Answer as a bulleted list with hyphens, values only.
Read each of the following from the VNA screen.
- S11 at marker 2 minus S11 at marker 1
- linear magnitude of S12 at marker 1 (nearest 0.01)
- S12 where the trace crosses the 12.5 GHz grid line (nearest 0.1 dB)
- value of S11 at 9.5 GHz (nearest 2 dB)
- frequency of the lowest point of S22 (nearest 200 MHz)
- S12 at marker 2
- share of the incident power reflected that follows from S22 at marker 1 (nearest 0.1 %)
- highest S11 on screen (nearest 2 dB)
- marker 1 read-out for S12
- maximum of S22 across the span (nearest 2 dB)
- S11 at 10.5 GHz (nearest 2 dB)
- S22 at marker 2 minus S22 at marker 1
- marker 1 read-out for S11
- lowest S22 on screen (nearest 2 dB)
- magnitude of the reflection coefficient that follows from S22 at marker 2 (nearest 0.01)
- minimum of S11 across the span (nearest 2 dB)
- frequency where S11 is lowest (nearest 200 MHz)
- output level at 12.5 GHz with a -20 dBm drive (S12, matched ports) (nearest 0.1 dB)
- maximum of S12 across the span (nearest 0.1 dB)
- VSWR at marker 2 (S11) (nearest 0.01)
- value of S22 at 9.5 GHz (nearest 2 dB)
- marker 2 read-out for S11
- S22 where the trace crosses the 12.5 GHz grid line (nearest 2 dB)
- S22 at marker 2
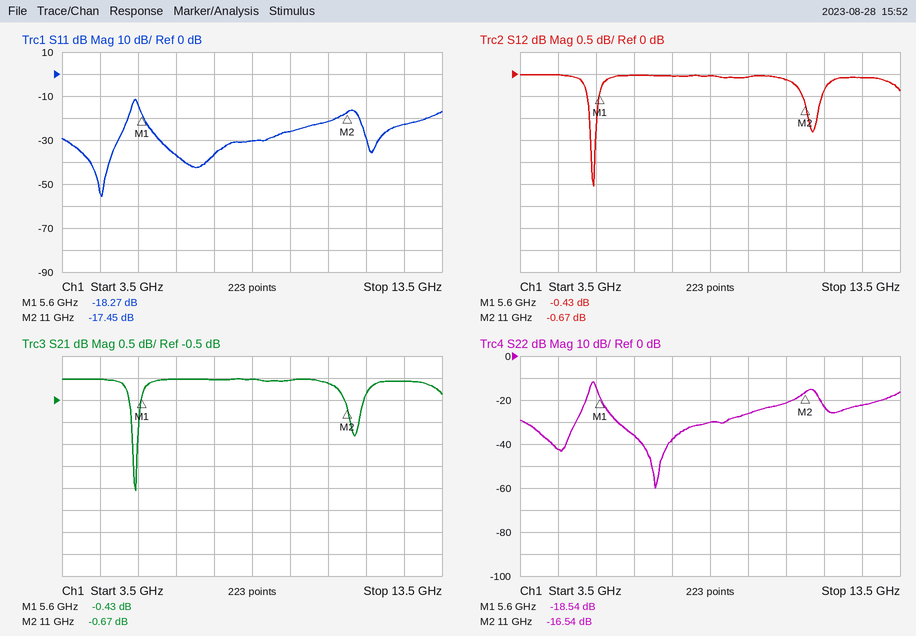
- 0.82 dB
- 0.95
- -0.1 dB
- -26 dB
- 7.0 GHz
- -0.67 dB
- 1.4 %
- -12 dB
- -0.43 dB
- -12 dB
- -22 dB
- 2.00 dB
- -18.27 dB
- -60 dB
- 0.15
- -56 dB
- 4.6 GHz
- -20.1 dBm
- 0.0 dB
- 1.31
- -26 dB
- -17.45 dB
- -22 dB
- -16.54 dB
